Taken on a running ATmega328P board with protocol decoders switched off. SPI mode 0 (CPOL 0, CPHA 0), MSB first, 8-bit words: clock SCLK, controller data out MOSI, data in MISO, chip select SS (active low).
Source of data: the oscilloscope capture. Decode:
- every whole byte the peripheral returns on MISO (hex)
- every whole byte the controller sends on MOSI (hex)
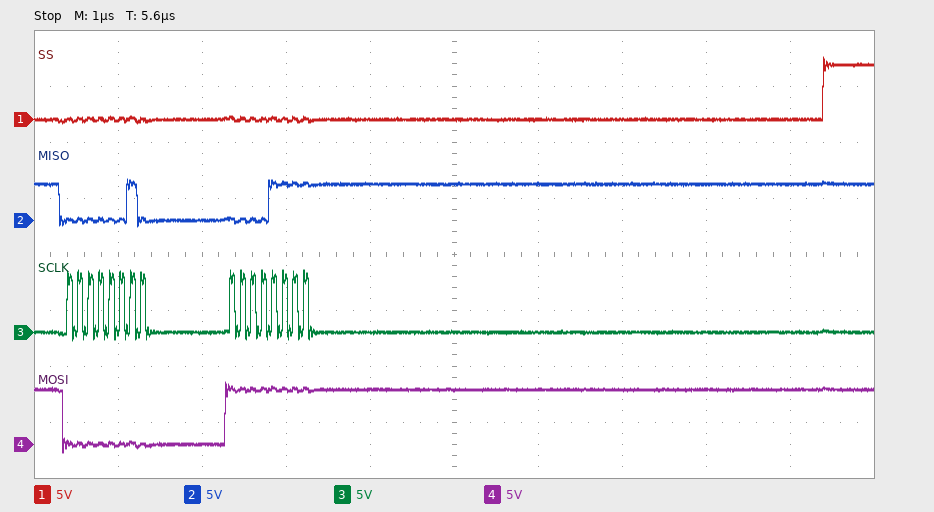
02 0F
00 FF
